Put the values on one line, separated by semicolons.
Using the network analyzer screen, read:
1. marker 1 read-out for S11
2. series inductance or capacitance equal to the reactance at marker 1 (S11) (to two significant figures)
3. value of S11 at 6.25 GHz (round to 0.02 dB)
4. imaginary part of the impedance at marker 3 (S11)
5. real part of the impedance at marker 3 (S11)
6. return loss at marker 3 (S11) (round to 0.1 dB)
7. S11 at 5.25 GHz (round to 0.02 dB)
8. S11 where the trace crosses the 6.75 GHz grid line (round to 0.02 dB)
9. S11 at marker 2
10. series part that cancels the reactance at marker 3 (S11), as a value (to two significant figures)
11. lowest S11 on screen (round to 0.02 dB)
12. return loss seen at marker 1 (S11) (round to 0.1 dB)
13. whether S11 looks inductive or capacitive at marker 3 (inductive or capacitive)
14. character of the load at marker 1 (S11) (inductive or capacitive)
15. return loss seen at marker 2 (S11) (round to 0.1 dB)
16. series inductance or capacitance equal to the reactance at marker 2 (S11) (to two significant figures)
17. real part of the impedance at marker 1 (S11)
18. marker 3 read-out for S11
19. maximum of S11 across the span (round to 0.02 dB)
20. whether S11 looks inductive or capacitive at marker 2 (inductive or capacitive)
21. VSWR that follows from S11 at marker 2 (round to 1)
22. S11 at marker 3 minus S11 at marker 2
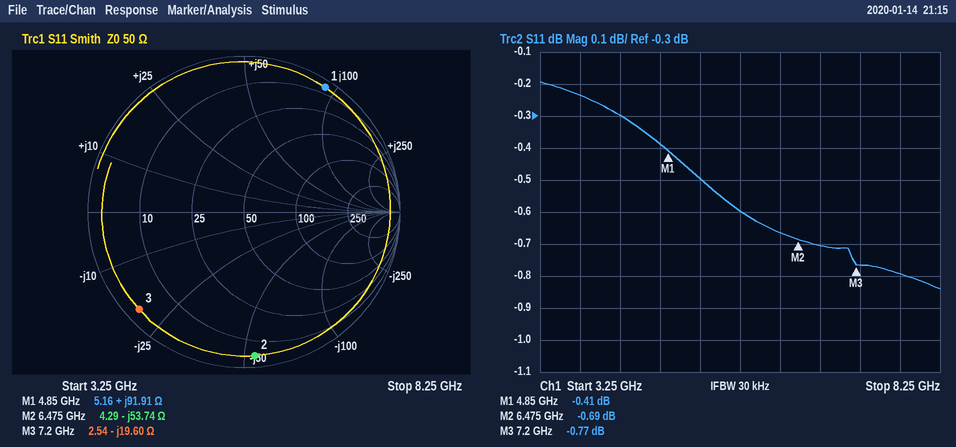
-0.41 dB; 3.0 nH; -0.66 dB; -19.60 Ω; 2.54 Ω; 0.8 dB; -0.50 dB; -0.70 dB; -0.69 dB; 430 pH; -0.84 dB; 0.4 dB; capacitive; inductive; 0.7 dB; 460 fF; 5.16 Ω; -0.77 dB; -0.20 dB; capacitive; 25; -0.08 dB
